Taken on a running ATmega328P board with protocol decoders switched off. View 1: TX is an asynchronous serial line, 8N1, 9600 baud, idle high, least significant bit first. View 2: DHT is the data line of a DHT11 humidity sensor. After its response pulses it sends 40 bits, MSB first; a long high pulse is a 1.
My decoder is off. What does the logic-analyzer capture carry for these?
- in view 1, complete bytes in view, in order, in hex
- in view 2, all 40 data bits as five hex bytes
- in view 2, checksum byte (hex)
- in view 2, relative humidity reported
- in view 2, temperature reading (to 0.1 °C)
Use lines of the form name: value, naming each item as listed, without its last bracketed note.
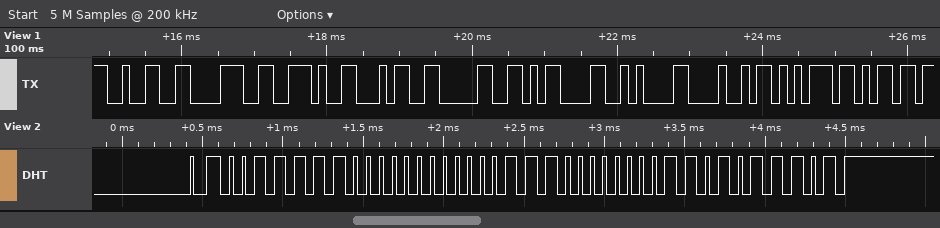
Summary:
in view 1, complete bytes in view, in order, in hex: 32 38 2E 34 30 0D 0A 48 75 6D
in view 2, all 40 data bits as five hex bytes: 3E 00 1C 03 5D
in view 2, checksum byte: 0x5D
in view 2, relative humidity reported: 62 %
in view 2, temperature reading: 28.3 °C
